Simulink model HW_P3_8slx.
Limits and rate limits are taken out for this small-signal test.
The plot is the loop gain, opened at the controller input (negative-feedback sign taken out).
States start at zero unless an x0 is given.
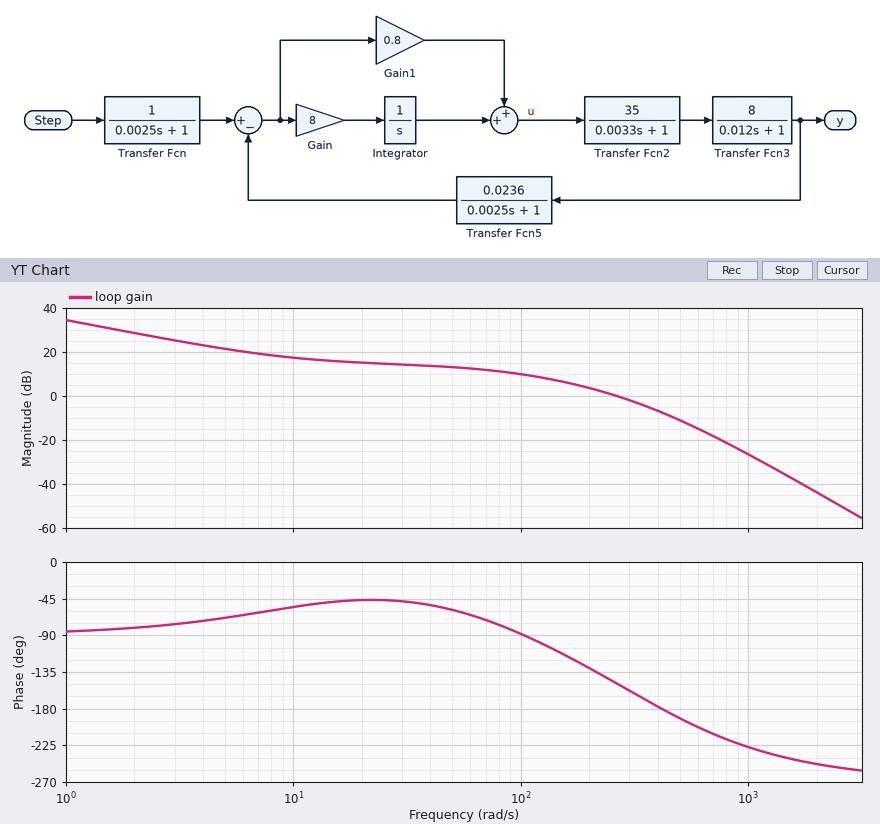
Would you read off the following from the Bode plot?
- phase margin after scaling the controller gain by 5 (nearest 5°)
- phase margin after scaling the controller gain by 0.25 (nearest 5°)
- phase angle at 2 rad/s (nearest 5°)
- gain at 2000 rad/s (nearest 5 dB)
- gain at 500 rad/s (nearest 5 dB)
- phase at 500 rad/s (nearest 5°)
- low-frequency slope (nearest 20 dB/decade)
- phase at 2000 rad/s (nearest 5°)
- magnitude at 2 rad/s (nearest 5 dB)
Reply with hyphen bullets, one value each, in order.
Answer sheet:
- -20°
- 110°
- -80°
- -45 dB
- -10 dB
- -190°
- -20 dB/decade
- -250°
- 30 dB
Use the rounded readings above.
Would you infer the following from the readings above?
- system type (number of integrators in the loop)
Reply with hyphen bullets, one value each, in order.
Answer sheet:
- 1
